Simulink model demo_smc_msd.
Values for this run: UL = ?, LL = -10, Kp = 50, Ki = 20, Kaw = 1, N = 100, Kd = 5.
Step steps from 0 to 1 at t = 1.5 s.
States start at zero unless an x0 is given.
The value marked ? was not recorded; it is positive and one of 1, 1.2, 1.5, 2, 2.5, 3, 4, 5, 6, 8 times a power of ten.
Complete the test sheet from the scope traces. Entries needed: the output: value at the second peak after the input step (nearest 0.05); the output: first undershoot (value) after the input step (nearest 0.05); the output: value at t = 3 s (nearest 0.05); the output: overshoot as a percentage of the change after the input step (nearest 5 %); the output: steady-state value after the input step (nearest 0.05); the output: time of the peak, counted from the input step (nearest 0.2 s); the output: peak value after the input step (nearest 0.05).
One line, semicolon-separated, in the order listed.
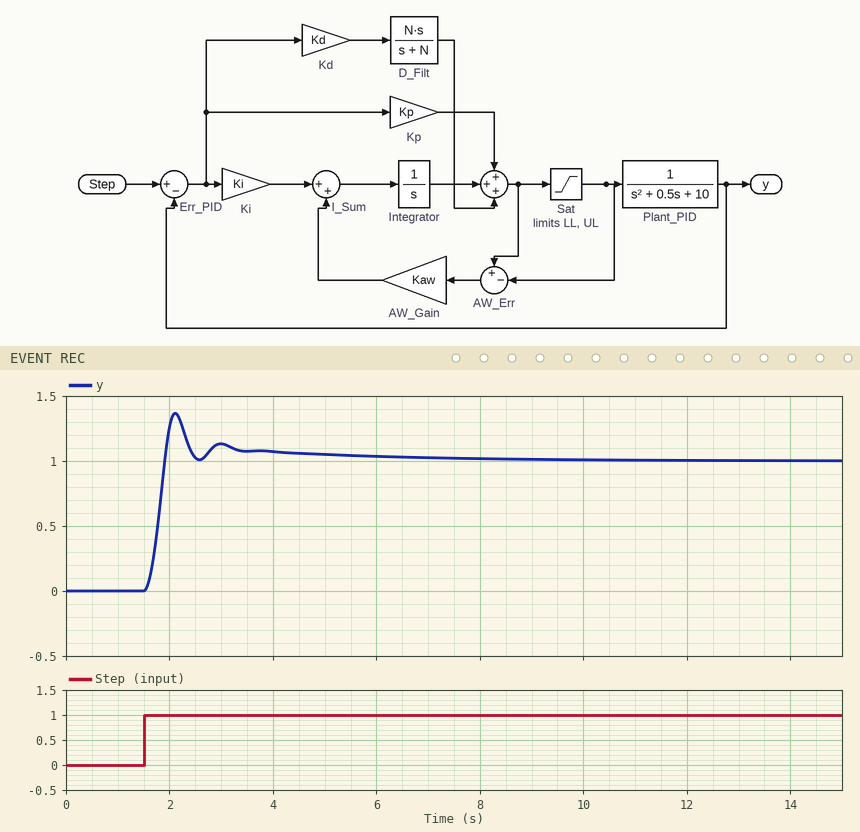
1.15; 1.00; 1.15; 35 %; 1.00; 0.6 s; 1.35
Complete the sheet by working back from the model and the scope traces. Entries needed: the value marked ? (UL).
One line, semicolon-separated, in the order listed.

15
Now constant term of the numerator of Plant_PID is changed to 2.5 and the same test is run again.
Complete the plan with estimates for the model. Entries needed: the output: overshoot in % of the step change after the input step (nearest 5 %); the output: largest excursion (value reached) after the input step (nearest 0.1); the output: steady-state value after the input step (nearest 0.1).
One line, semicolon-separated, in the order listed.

25 %; 1.2; 1.0
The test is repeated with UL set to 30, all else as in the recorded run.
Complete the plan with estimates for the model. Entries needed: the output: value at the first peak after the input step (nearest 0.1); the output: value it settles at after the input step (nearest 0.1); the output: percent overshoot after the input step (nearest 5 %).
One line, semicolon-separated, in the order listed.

1.3; 1.0; 30 %
